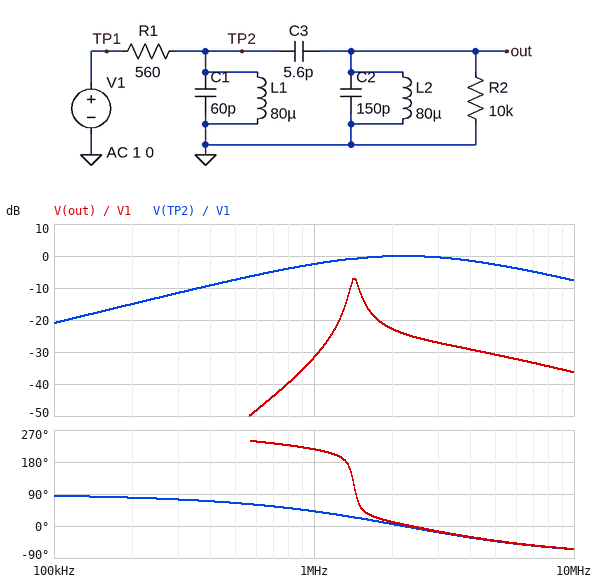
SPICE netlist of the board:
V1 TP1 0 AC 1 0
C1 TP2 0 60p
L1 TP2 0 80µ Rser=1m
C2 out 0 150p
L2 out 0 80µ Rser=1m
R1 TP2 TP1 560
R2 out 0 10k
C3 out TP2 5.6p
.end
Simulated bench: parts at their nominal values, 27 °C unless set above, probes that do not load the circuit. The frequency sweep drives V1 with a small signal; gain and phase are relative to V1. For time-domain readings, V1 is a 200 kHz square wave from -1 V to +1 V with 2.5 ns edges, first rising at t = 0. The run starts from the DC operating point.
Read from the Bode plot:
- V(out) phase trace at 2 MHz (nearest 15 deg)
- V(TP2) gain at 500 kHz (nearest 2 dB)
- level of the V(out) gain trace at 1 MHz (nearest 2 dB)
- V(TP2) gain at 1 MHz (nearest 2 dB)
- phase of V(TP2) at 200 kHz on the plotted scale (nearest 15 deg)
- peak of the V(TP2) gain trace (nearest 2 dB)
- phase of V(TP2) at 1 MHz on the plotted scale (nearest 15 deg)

15 deg
-8 dB
-32 dB
-2 dB
75 deg
0 dB
45 deg
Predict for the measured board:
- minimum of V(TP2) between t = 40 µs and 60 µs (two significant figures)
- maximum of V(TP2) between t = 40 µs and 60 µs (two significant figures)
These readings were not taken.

-1.5 V
1.5 V
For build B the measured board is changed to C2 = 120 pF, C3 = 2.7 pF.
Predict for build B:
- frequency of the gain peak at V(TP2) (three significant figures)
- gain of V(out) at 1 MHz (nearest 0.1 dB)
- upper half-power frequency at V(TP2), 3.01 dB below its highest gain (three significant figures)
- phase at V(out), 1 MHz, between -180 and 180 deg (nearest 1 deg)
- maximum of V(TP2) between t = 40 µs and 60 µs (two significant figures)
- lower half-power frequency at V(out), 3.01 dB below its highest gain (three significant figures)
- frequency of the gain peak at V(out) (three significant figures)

2.25 MHz
-39.7 dB
5.46 MHz
-143 deg
1.5 V
1.55 MHz
1.61 MHz
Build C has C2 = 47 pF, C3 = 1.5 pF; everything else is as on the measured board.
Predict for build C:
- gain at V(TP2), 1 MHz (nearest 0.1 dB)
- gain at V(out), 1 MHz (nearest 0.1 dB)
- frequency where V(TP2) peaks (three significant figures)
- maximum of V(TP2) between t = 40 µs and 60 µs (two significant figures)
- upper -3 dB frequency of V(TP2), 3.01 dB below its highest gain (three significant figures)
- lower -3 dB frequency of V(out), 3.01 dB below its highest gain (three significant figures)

-2.6 dB
-47.6 dB
2.25 MHz
1.5 V
5.56 MHz
2.41 MHz
